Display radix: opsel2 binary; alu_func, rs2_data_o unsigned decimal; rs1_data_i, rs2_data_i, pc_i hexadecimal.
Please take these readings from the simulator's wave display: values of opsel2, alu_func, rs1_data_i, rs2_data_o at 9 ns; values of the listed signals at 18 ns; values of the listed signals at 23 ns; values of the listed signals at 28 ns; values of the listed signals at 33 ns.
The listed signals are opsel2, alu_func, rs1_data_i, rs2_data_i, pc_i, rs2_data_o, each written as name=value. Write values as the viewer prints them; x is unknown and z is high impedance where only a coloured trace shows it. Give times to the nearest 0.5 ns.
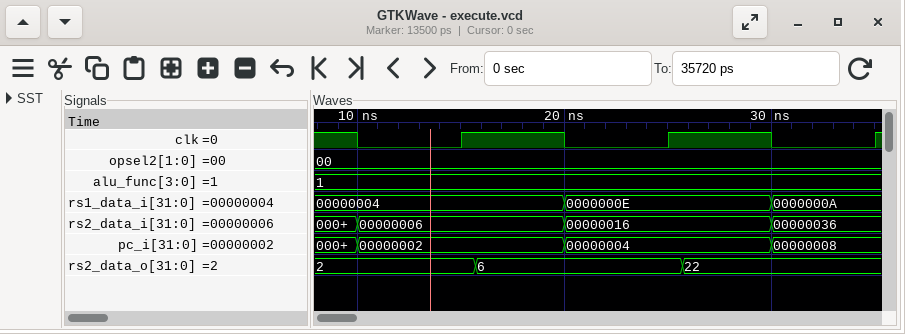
opsel2=00, alu_func=1, rs1_data_i=00000004, rs2_data_o=2
opsel2=00, alu_func=1, rs1_data_i=00000004, rs2_data_i=00000006, pc_i=00000002, rs2_data_o=6
opsel2=00, alu_func=1, rs1_data_i=0000000E, rs2_data_i=00000016, pc_i=00000004, rs2_data_o=6
opsel2=00, alu_func=1, rs1_data_i=0000000E, rs2_data_i=00000016, pc_i=00000004, rs2_data_o=22
opsel2=00, alu_func=1, rs1_data_i=0000000A, rs2_data_i=00000036, pc_i=00000008, rs2_data_o=22
